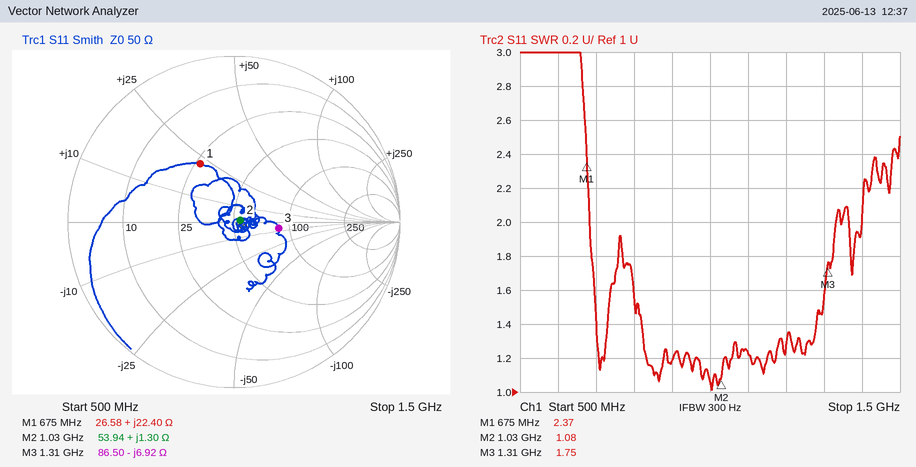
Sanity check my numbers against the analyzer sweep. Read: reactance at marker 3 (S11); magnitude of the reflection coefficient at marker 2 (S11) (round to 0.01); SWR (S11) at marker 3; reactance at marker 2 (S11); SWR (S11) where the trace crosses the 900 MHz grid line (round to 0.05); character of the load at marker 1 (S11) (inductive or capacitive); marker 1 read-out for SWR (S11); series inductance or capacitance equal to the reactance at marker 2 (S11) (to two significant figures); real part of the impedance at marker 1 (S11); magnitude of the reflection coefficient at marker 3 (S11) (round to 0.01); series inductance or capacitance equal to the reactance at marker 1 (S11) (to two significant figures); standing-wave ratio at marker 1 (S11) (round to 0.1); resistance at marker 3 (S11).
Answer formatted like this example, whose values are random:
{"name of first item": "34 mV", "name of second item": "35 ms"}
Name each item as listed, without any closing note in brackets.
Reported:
{"reactance at marker 3": "-6.92 Ω", "magnitude of the reflection coefficient at marker 2 (S11)": "0.04", "SWR (S11) at marker 3": "1.75", "reactance at marker 2": "+1.30 Ω", "SWR (S11) where the trace crosses the 900 MHz grid line": "1.20", "character of the load at marker 1 (S11)": "inductive", "marker 1 read-out for SWR": "2.37", "series inductance or capacitance equal to the reactance at marker 2 (S11)": "200 pH", "real part of the impedance at marker 1": "26.58 Ω", "magnitude of the reflection coefficient at marker 3 (S11)": "0.27", "series inductance or capacitance equal to the reactance at marker 1 (S11)": "5.3 nH", "standing-wave ratio at marker 1 (S11)": "2.4", "resistance at marker 3": "86.50 Ω"}
